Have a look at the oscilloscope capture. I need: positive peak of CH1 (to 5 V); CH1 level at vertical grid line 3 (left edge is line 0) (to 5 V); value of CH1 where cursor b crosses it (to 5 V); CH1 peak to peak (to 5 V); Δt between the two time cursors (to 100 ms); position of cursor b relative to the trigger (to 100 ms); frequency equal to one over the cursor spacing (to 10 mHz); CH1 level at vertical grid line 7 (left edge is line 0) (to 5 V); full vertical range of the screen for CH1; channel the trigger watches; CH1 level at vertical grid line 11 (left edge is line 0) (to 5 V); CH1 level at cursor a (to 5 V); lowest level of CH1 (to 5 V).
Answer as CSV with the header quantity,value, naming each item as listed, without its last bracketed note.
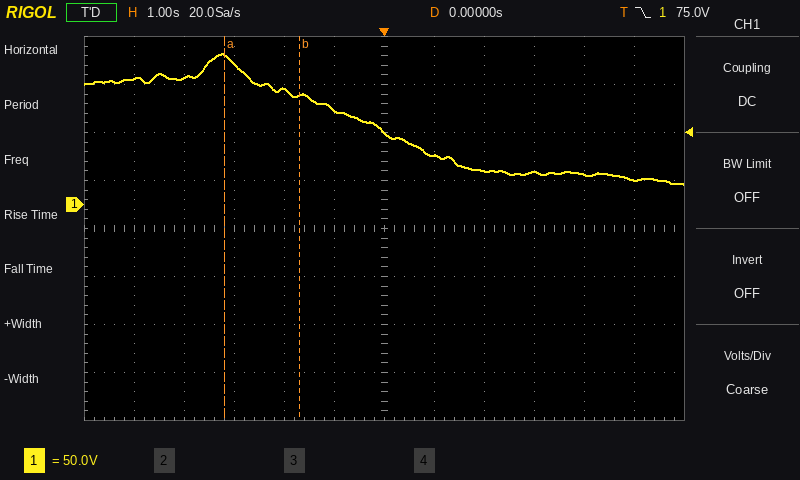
quantity,value
positive peak of CH1,155 V
CH1 level at vertical grid line 3 (left edge is line 0),145 V
value of CH1 where cursor b crosses it,115 V
CH1 peak to peak,135 V
Δt between the two time cursors,1.5 s
position of cursor b relative to the trigger,-1.7 s
frequency equal to one over the cursor spacing,670 mHz
CH1 level at vertical grid line 7 (left edge is line 0),50 V
full vertical range of the screen for CH1,400 V
channel the trigger watches,CH1
CH1 level at vertical grid line 11 (left edge is line 0),25 V
CH1 level at cursor a,155 V
lowest level of CH1,20 V
